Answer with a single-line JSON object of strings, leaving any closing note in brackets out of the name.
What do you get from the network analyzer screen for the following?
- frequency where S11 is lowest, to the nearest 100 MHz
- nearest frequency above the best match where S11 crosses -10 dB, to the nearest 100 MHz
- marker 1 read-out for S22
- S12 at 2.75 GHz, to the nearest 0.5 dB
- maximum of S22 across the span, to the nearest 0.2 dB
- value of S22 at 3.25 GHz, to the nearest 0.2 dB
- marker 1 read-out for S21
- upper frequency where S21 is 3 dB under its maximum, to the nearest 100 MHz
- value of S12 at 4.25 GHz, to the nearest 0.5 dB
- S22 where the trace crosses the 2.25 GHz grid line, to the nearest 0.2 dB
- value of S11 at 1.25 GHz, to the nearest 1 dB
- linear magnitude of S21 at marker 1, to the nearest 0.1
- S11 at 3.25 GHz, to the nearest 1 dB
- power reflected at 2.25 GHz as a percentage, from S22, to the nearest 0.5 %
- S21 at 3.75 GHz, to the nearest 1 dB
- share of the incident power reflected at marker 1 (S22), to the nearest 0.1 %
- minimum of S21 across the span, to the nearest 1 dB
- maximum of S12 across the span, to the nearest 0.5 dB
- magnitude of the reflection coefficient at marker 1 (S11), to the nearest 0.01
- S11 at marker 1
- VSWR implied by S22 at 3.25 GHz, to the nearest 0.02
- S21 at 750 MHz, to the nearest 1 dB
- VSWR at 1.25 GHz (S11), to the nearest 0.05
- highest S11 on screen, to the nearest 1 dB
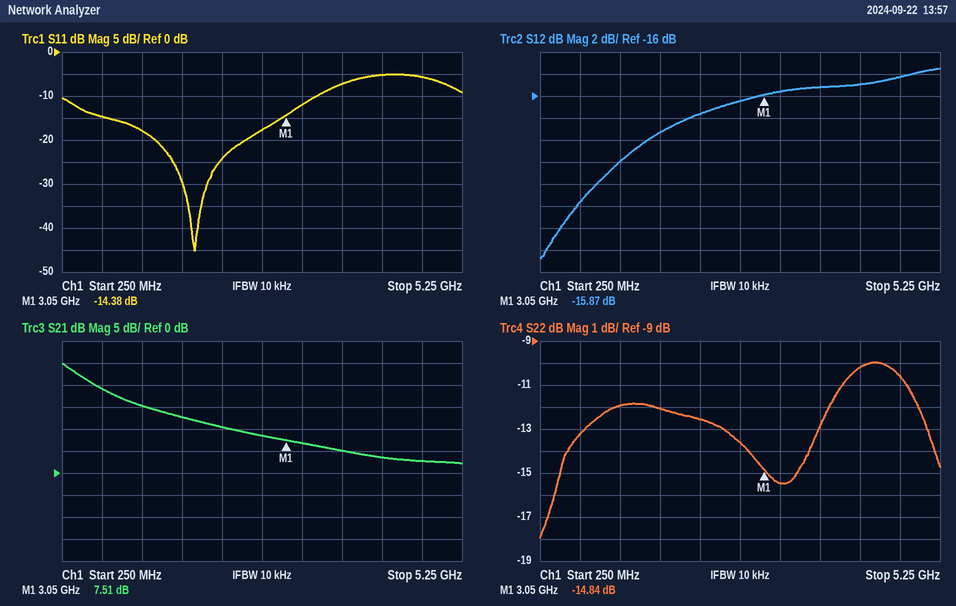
{"frequency where S11 is lowest, to the nearest 100 MHz": "1.9 GHz", "nearest frequency above the best match where S11 crosses -10 dB, to the nearest 100 MHz": "3.4 GHz", "marker 1 read-out for S22": "-14.84 dB", "S12 at 2.75 GHz, to the nearest 0.5 dB": "-16.5 dB", "maximum of S22 across the span, to the nearest 0.2 dB": "-10.0 dB", "value of S22 at 3.25 GHz, to the nearest 0.2 dB": "-15.4 dB", "marker 1 read-out for S21": "7.51 dB", "upper frequency where S21 is 3 dB under its maximum, to the nearest 100 MHz": "500 MHz", "value of S12 at 4.25 GHz, to the nearest 0.5 dB": "-15.0 dB", "S22 where the trace crosses the 2.25 GHz grid line, to the nearest 0.2 dB": "-12.6 dB", "value of S11 at 1.25 GHz, to the nearest 1 dB": "-18 dB", "linear magnitude of S21 at marker 1, to the nearest 0.1": "2.4", "S11 at 3.25 GHz, to the nearest 1 dB": "-12 dB", "power reflected at 2.25 GHz as a percentage, from S22, to the nearest 0.5 %": "5.5 %", "S21 at 3.75 GHz, to the nearest 1 dB": "5 dB", "share of the incident power reflected at marker 1 (S22), to the nearest 0.1 %": "3.3 %", "minimum of S21 across the span, to the nearest 1 dB": "2 dB", "maximum of S12 across the span, to the nearest 0.5 dB": "-13.5 dB", "magnitude of the reflection coefficient at marker 1 (S11), to the nearest 0.01": "0.19", "S11 at marker 1": "-14.38 dB", "VSWR implied by S22 at 3.25 GHz, to the nearest 0.02": "1.40", "S21 at 750 MHz, to the nearest 1 dB": "19 dB", "VSWR at 1.25 GHz (S11), to the nearest 0.05": "1.30", "highest S11 on screen, to the nearest 1 dB": "-5 dB"}
